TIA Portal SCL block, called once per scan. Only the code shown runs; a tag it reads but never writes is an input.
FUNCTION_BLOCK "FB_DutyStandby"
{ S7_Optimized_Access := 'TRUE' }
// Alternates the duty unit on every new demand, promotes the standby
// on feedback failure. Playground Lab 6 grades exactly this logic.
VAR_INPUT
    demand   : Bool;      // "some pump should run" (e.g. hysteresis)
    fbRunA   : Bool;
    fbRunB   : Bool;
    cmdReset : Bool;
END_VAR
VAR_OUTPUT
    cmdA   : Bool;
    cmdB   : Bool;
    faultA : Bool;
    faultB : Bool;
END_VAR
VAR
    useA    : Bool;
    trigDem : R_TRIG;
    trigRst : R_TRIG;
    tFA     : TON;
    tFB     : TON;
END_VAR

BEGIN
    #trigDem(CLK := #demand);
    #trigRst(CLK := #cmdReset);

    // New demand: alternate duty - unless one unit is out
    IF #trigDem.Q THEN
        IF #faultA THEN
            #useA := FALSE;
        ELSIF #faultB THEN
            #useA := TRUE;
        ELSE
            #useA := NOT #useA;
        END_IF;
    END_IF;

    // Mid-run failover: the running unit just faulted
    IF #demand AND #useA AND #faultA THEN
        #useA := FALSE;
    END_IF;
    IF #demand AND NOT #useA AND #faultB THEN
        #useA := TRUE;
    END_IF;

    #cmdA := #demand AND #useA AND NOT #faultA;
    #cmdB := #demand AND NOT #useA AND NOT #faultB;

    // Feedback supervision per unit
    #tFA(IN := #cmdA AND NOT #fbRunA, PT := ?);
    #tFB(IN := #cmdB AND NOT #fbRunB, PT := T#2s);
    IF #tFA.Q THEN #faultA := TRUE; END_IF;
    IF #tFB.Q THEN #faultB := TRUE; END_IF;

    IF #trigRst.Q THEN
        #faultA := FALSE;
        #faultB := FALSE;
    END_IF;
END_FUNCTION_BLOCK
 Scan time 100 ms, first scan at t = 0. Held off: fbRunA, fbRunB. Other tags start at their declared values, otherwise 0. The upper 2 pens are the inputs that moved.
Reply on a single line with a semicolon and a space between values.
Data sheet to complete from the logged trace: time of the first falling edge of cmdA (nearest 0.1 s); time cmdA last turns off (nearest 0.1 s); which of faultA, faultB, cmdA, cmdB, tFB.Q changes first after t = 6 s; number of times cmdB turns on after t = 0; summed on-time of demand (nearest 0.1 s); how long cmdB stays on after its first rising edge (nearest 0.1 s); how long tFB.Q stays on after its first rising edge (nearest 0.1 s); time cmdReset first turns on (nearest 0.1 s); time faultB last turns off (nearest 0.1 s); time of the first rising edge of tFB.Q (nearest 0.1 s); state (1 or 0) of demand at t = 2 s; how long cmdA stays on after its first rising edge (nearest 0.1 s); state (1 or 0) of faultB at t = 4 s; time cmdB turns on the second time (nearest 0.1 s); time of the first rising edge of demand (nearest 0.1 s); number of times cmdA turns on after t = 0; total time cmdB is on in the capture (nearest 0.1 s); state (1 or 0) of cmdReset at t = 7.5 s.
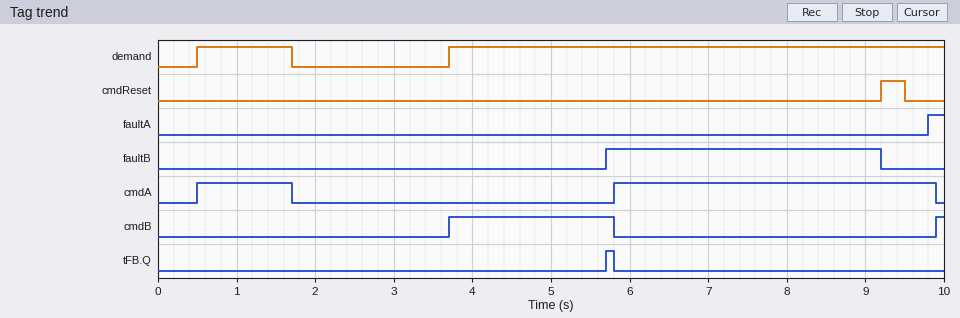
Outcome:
1.7 s; 9.9 s; faultB; 2; 7.5 s; 2.1 s; 0.1 s; 9.2 s; 9.2 s; 5.7 s; 0; 1.2 s; 0; 9.9 s; 0.5 s; 2; 2.2 s; 0
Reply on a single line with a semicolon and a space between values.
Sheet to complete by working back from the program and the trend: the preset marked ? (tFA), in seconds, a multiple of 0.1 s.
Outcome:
4.0 s
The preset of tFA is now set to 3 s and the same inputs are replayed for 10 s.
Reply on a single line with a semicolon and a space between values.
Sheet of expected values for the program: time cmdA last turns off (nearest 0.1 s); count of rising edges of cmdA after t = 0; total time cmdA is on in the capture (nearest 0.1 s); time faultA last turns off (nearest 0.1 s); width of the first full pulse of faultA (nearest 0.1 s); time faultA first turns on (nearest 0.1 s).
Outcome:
8.9 s; 3; 5.0 s; 9.2 s; 0.4 s; 8.8 s
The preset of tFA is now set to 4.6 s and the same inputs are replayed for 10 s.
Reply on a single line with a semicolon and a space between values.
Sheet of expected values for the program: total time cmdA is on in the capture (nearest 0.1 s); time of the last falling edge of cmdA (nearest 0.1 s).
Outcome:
5.4 s; 1.7 s
